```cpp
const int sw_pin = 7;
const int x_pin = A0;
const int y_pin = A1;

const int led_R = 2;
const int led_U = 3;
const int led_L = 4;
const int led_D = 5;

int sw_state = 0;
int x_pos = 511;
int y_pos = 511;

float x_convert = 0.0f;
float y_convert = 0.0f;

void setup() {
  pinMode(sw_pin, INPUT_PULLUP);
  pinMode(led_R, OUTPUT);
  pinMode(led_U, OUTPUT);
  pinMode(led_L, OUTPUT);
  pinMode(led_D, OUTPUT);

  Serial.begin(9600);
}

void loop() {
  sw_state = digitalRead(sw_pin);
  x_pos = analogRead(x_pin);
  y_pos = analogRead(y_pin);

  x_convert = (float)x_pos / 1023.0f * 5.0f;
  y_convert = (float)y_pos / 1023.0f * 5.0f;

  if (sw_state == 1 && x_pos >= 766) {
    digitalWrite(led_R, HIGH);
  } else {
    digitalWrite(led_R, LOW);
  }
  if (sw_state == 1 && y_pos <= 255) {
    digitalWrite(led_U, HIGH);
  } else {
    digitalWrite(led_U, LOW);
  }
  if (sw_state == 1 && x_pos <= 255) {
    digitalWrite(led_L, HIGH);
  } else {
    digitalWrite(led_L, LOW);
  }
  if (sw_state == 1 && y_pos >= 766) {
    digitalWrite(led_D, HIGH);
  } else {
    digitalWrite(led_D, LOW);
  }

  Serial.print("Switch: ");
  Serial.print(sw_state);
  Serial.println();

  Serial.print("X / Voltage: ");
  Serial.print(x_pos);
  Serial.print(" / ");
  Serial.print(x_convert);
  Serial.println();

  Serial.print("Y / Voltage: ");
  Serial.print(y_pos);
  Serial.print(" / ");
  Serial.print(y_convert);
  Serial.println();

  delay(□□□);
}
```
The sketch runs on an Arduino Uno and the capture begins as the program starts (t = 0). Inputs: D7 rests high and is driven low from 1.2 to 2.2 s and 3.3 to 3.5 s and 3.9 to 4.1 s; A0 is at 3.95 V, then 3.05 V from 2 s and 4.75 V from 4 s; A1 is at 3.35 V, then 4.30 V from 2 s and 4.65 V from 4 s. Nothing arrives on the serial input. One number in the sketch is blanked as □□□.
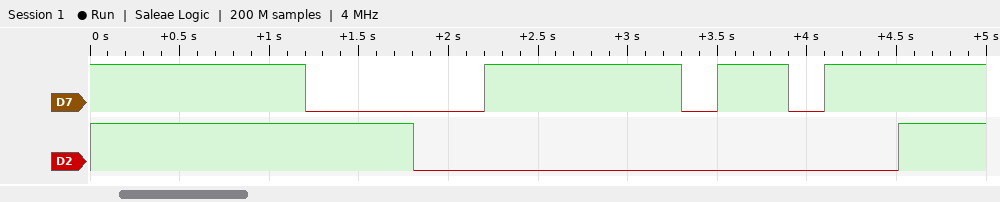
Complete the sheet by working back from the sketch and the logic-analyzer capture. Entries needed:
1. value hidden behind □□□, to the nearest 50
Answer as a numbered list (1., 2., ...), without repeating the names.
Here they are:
1. 900
